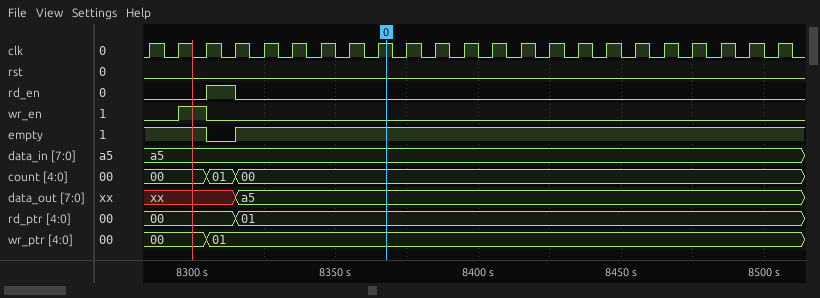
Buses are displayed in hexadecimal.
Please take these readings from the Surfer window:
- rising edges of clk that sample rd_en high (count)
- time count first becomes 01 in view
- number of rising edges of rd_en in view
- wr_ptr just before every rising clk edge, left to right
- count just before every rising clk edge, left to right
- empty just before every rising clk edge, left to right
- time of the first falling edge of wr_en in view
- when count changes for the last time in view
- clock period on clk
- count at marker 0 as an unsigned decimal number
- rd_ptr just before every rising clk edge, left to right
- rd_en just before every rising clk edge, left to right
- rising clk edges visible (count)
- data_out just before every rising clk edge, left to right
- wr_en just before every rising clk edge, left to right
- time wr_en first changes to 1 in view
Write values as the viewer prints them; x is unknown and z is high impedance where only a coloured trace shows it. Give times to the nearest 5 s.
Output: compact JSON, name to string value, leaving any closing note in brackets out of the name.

{"rising edges of clk that sample rd_en high": "1", "time count first becomes 01 in view": "8305 s", "number of rising edges of rd_en in view": "1", "wr_ptr just before every rising clk edge, left to right": "00, 00, 00, 01, 01, 01, 01, 01, 01, 01, 01, 01, 01, 01, 01, 01, 01, 01, 01, 01, 01, 01, 01", "count just before every rising clk edge, left to right": "00, 00, 00, 01, 00, 00, 00, 00, 00, 00, 00, 00, 00, 00, 00, 00, 00, 00, 00, 00, 00, 00, 00", "empty just before every rising clk edge, left to right": "1 1 1 0 1 1 1 1 1 1 1 1 1 1 1 1 1 1 1 1 1 1 1", "time of the first falling edge of wr_en in view": "8305 s", "when count changes for the last time in view": "8315 s", "clock period on clk": "10 s", "count at marker 0 as an unsigned decimal number": "0", "rd_ptr just before every rising clk edge, left to right": "00, 00, 00, 00, 01, 01, 01, 01, 01, 01, 01, 01, 01, 01, 01, 01, 01, 01, 01, 01, 01, 01, 01", "rd_en just before every rising clk edge, left to right": "0 0 0 1 0 0 0 0 0 0 0 0 0 0 0 0 0 0 0 0 0 0 0", "rising clk edges visible": "23", "data_out just before every rising clk edge, left to right": "xx, xx, xx, xx, a5, a5, a5, a5, a5, a5, a5, a5, a5, a5, a5, a5, a5, a5, a5, a5, a5, a5, a5", "wr_en just before every rising clk edge, left to right": "0 0 1 0 0 0 0 0 0 0 0 0 0 0 0 0 0 0 0 0 0 0 0", "time wr_en first changes to 1 in view": "8295 s"}
